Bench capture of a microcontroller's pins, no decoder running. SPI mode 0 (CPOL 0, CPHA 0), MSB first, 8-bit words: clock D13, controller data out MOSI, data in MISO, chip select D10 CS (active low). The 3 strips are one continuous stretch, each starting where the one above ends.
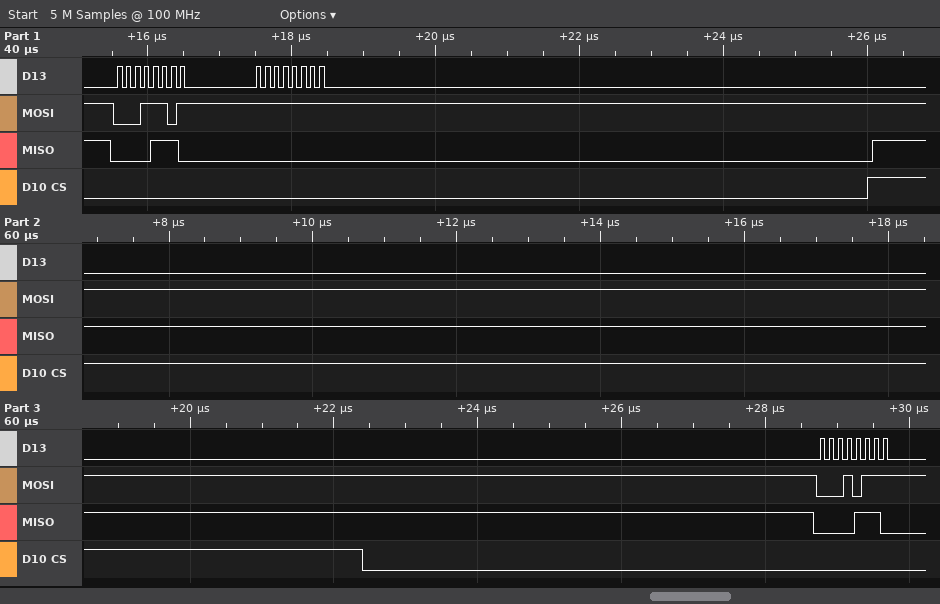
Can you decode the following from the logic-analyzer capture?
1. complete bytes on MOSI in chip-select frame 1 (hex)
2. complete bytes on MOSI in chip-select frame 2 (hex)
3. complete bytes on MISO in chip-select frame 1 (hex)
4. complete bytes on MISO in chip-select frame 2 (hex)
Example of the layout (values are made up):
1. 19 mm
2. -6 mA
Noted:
1. 1D FF
2. 17
3. 0E 00
4. 0E
